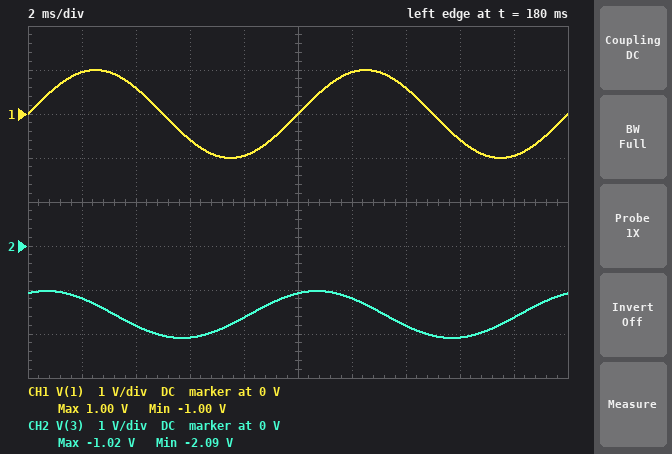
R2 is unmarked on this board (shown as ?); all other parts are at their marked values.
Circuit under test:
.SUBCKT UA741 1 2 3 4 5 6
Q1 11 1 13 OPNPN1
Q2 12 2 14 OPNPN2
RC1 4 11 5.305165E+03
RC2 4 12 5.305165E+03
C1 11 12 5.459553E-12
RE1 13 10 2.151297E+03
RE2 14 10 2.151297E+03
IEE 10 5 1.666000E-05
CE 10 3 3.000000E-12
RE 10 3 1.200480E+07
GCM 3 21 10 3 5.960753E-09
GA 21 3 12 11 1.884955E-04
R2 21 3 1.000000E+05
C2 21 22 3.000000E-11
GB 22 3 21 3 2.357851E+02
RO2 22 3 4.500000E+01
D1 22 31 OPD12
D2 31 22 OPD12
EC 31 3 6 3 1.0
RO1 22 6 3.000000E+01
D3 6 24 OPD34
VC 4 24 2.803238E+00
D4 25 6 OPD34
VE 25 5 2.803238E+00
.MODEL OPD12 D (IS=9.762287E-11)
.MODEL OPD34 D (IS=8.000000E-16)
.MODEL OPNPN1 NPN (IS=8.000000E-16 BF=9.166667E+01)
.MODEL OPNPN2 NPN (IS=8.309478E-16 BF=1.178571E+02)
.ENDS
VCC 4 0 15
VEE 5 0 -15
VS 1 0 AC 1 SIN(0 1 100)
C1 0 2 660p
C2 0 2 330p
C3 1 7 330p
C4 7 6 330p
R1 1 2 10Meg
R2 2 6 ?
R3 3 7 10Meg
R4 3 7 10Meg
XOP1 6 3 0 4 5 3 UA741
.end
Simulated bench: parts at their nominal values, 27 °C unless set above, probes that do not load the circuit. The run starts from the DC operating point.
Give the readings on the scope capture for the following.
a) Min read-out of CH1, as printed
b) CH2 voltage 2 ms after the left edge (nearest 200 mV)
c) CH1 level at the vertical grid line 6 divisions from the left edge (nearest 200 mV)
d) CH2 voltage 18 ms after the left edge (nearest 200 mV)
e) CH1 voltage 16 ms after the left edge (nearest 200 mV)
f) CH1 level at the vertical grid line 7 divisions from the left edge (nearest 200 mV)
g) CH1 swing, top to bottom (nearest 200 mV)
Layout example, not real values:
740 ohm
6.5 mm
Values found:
-1.00 V
-1.2 V
1.0 V
-1.6 V
-600 mV
600 mV
2.0 V
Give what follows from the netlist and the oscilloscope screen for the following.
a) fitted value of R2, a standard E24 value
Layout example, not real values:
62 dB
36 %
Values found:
7.5 MΩ
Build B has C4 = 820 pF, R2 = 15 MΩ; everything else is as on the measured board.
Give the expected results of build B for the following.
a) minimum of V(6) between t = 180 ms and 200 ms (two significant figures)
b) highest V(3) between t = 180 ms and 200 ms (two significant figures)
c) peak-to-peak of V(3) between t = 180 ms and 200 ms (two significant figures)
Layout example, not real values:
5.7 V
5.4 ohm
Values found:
-3.1 V
-1.3 V
1.8 V
